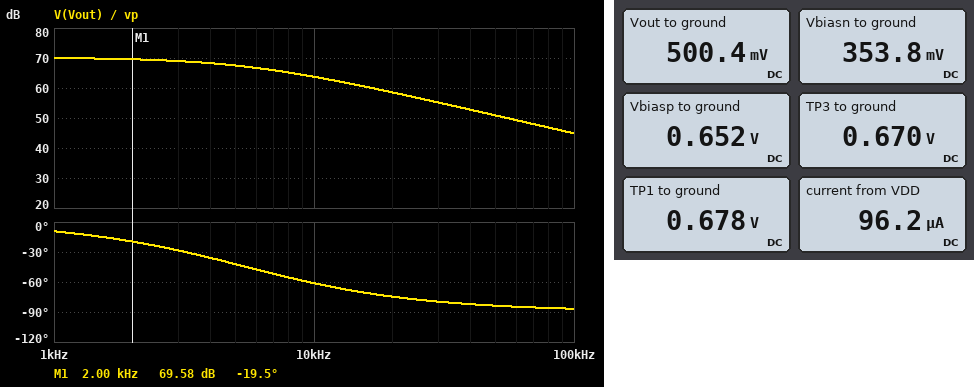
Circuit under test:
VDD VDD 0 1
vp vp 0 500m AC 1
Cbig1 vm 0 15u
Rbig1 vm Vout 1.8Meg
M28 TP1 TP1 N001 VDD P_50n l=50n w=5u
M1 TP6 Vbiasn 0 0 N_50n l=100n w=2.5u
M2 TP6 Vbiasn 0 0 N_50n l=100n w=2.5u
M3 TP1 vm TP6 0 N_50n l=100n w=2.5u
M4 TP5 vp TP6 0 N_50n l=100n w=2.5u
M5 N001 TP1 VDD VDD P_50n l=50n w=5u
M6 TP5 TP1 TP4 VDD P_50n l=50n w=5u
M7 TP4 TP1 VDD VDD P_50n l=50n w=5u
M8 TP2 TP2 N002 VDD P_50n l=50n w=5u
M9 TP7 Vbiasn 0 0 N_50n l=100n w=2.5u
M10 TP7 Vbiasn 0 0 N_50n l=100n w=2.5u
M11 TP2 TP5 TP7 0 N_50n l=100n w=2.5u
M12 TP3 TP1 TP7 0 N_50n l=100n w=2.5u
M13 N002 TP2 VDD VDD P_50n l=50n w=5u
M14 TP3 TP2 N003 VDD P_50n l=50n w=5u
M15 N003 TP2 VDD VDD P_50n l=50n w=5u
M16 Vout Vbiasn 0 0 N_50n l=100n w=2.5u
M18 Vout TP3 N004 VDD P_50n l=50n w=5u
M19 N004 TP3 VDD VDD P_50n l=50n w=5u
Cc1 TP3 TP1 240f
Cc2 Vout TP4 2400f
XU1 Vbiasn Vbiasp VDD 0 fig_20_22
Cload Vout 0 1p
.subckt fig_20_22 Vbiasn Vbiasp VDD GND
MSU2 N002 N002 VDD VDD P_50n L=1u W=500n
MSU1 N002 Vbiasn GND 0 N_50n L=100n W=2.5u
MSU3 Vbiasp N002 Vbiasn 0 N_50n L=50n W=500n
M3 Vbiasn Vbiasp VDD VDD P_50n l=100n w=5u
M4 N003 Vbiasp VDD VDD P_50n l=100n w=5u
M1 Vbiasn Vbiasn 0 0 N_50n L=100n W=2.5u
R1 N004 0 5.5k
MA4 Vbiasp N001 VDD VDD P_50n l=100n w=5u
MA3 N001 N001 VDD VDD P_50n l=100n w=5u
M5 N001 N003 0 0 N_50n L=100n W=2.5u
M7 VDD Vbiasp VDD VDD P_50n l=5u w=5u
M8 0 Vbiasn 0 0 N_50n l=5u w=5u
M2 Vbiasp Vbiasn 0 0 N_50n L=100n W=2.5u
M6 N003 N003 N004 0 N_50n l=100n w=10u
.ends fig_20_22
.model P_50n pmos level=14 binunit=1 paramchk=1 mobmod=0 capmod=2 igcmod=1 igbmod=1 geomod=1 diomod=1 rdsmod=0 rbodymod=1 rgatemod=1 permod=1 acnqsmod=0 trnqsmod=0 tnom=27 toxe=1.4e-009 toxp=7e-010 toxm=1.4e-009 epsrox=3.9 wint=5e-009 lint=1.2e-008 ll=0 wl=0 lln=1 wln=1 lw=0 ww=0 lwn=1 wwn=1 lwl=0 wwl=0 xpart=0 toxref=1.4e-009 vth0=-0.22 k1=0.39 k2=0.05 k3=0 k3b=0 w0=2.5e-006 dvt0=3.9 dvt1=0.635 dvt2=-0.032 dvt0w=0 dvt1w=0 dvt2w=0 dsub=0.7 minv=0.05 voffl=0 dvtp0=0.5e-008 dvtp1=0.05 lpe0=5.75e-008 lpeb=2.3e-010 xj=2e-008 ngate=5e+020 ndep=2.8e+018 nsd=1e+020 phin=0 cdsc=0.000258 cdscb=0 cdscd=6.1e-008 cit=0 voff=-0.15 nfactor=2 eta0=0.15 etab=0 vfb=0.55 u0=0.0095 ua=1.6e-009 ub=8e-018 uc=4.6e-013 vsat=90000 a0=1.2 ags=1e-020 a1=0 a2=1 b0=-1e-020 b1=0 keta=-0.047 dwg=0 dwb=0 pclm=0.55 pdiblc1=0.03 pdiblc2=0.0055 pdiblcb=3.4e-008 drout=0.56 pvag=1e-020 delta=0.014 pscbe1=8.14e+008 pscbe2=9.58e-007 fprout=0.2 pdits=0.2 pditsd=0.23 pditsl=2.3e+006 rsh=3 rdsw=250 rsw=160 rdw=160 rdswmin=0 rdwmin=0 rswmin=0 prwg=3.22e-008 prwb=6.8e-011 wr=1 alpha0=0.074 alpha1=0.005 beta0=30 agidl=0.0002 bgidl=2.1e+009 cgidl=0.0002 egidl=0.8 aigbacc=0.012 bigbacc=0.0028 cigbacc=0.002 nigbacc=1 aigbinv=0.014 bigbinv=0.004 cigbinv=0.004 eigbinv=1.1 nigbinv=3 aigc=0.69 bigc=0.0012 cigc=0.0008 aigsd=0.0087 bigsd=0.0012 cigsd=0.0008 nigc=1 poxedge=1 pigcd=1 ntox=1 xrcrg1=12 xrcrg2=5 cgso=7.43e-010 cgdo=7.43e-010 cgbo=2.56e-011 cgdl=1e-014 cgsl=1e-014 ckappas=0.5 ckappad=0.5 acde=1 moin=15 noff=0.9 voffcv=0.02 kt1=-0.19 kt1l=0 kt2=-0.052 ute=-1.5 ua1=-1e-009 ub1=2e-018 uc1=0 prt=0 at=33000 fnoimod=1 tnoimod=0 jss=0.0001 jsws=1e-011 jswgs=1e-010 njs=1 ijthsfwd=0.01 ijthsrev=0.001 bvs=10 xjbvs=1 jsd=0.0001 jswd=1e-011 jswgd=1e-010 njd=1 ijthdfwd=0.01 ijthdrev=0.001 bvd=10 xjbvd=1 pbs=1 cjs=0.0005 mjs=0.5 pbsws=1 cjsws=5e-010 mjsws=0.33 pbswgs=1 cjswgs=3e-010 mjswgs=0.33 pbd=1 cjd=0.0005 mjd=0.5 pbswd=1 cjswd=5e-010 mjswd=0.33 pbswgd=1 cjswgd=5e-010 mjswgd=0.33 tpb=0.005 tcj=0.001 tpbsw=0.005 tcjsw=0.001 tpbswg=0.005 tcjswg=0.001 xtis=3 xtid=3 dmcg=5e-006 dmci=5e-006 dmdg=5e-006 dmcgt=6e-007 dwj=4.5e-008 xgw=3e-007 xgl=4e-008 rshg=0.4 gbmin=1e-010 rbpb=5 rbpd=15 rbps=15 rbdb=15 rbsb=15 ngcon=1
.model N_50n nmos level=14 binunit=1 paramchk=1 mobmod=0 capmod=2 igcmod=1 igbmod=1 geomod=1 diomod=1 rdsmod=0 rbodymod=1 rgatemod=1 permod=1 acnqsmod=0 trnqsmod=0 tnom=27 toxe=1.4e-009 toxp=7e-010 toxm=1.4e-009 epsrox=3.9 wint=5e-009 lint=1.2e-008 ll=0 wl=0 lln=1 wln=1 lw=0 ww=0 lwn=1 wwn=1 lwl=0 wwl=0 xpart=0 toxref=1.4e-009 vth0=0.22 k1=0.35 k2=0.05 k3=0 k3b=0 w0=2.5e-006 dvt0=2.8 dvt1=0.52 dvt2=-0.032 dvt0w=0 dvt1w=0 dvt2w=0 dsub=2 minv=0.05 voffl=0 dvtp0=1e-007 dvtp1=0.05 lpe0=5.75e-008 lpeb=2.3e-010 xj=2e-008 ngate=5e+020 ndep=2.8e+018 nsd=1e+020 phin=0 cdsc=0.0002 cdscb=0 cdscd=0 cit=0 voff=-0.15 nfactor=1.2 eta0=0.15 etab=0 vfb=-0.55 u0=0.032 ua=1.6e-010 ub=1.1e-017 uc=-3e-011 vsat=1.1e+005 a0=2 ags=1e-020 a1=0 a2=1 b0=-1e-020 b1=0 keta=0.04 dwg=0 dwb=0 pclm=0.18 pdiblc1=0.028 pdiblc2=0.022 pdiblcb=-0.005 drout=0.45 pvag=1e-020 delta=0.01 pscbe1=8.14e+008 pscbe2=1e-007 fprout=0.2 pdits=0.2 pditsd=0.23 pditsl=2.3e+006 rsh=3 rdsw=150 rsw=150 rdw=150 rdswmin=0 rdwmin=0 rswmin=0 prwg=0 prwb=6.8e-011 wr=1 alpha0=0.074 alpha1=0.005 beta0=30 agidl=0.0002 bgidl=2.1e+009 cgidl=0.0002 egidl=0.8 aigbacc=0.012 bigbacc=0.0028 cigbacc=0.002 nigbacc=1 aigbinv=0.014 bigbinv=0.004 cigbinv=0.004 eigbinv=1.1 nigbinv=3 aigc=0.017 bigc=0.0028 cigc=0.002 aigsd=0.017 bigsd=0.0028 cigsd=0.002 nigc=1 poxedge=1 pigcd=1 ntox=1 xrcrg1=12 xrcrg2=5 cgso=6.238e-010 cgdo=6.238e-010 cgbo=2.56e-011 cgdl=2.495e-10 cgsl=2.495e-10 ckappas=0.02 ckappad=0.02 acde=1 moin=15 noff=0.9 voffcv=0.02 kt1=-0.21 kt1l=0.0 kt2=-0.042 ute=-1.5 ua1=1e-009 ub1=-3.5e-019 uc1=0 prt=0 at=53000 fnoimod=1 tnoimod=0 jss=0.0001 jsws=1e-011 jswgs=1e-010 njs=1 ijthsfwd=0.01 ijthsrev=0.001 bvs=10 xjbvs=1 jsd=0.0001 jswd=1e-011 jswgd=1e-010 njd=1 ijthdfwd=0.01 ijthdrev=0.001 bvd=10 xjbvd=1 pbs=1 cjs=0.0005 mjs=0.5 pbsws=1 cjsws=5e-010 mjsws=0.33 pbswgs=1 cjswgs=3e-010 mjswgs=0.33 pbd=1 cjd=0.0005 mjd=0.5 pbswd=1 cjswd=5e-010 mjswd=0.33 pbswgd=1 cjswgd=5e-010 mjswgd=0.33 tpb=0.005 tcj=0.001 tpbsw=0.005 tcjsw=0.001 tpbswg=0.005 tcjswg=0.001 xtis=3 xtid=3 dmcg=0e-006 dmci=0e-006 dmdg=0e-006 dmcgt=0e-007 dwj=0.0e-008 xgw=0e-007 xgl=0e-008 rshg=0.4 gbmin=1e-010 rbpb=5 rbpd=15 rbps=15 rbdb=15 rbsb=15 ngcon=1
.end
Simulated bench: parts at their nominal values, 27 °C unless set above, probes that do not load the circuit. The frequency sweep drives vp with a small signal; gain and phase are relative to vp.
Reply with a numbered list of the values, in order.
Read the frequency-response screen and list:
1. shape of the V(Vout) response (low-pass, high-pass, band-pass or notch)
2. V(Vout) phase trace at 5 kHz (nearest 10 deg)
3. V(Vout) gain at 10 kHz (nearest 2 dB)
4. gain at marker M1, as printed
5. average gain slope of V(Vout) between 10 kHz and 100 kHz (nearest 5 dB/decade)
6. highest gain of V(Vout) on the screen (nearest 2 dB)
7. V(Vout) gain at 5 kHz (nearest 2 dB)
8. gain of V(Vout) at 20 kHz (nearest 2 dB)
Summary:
1. low-pass
2. -40 deg
3. 64 dB
4. 69.58 dB
5. -20 dB/decade
6. 70 dB
7. 68 dB
8. 58 dB
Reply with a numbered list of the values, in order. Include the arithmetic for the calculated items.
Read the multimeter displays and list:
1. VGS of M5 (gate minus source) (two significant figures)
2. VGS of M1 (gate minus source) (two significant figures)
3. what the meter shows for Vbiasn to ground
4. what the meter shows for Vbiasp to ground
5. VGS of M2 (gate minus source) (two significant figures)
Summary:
1. 678 mV - 1 V = -320 mV
2. 353.8 mV = 350 mV
3. 353.8 mV
4. 0.652 V
5. 353.8 mV = 350 mV
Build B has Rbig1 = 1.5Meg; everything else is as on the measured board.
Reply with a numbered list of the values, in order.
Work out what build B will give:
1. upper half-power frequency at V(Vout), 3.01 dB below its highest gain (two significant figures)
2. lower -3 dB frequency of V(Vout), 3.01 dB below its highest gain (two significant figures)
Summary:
1. 5.6 kHz
2. 22 Hz
